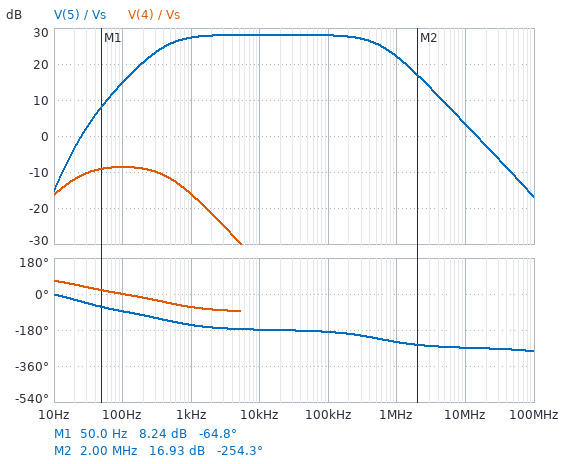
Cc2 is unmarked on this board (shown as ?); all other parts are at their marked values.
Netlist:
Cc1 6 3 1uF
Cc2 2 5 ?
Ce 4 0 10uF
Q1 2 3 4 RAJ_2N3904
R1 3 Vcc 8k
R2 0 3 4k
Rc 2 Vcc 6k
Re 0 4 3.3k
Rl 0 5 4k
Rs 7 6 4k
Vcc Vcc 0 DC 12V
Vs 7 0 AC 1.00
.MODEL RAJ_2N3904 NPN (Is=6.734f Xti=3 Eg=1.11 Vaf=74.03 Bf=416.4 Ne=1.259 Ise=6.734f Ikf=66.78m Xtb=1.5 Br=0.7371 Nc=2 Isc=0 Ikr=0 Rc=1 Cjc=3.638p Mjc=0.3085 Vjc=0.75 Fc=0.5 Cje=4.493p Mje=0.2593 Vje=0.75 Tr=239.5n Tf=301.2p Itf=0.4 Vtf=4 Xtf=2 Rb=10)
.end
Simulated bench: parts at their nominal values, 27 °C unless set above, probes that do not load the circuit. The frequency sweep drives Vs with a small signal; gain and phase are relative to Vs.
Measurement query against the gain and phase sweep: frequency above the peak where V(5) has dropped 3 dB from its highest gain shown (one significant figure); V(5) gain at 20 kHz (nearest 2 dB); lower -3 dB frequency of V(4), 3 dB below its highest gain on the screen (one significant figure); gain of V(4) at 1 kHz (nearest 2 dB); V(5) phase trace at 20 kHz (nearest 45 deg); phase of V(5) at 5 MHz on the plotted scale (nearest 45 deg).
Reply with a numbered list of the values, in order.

1. 600 kHz
2. 28 dB
3. 20 Hz
4. -16 dB
5. -180 deg
6. -270 deg
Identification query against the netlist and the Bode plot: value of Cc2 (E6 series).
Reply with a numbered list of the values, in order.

1. 1.5 µF
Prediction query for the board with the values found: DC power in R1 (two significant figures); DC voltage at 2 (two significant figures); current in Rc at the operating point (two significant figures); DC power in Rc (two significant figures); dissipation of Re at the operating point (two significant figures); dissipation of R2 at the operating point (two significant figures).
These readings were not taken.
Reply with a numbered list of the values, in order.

1. 8.0 mW
2. 6.0 V
3. 1.0 mA
4. 6.0 mW
5. 3.3 mW
6. 4.0 mW
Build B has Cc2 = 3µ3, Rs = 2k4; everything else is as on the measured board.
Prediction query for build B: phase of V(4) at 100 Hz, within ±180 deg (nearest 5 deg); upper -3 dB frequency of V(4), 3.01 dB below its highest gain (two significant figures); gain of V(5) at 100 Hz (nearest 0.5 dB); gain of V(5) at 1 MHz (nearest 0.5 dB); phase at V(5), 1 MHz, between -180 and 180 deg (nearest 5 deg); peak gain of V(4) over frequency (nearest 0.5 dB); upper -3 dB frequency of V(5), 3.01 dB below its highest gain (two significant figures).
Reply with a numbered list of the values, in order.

1. 5 deg
2. 520 Hz
3. 17.0 dB
4. 26.0 dB
5. 125 deg
6. -6.5 dB
7. 680 kHz
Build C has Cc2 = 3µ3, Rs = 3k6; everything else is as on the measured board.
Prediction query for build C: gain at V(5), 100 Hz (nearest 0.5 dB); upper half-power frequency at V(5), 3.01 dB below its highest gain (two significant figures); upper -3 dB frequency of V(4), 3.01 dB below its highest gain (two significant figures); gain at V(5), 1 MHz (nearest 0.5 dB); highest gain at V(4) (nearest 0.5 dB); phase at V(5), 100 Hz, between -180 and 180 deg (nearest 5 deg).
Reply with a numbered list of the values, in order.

1. 15.5 dB
2. 590 kHz
3. 490 Hz
4. 23.0 dB
5. -8.0 dB
6. -90 deg
